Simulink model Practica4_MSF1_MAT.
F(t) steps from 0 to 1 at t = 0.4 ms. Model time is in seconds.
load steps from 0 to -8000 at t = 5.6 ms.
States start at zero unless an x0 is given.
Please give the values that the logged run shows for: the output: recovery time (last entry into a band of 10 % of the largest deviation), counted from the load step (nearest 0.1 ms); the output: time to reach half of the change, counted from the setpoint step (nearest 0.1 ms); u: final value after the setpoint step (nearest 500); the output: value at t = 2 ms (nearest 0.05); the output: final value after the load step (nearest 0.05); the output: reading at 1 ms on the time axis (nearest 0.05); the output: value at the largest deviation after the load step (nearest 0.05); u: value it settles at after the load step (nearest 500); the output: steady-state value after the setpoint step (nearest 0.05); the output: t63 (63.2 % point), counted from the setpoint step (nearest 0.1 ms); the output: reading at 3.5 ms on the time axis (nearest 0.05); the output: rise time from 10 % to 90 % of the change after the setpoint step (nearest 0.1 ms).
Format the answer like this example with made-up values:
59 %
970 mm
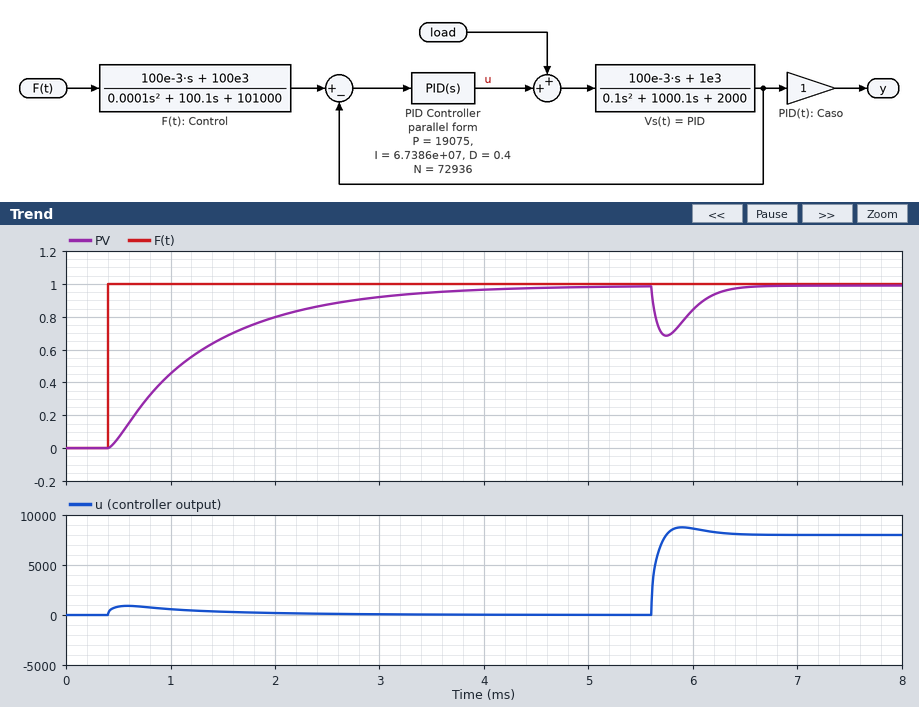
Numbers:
0.7 ms
0.7 ms
0
0.80
1.00
0.45
0.70
8000
1.00
1.0 ms
0.95
2.1 ms
